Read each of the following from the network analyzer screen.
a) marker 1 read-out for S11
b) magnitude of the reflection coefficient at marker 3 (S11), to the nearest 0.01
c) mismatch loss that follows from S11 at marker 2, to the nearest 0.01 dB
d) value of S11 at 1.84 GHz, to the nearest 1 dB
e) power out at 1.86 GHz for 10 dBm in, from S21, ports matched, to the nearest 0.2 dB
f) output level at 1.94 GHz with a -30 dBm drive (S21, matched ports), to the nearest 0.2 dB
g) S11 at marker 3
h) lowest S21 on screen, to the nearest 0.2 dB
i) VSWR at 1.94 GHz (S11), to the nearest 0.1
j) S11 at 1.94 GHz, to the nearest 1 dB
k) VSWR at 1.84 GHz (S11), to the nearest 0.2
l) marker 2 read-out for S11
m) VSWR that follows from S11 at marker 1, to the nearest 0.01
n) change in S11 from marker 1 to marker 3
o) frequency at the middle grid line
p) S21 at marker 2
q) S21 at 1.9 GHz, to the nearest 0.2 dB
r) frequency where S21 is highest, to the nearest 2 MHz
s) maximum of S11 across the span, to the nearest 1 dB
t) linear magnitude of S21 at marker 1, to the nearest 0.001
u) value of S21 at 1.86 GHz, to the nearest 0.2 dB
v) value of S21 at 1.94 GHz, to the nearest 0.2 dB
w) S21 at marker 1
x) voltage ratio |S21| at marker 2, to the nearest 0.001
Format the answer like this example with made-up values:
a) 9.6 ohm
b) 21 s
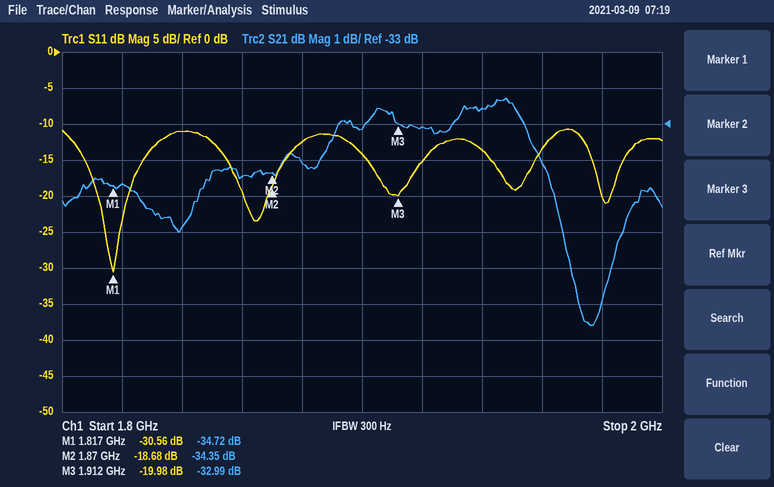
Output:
a) -30.56 dB
b) 0.10
c) 0.06 dB
d) -11 dB
e) -24.4 dBm
f) -62.6 dBm
g) -19.98 dB
h) -38.6 dB
i) 1.5
j) -14 dB
k) 1.8
l) -18.68 dB
m) 1.06
n) 10.58 dB
o) 1.9 GHz
p) -34.35 dB
q) -33.2 dB
r) 1.948 GHz
s) -11 dB
t) 0.018
u) -34.4 dB
v) -32.6 dB
w) -34.72 dB
x) 0.019
